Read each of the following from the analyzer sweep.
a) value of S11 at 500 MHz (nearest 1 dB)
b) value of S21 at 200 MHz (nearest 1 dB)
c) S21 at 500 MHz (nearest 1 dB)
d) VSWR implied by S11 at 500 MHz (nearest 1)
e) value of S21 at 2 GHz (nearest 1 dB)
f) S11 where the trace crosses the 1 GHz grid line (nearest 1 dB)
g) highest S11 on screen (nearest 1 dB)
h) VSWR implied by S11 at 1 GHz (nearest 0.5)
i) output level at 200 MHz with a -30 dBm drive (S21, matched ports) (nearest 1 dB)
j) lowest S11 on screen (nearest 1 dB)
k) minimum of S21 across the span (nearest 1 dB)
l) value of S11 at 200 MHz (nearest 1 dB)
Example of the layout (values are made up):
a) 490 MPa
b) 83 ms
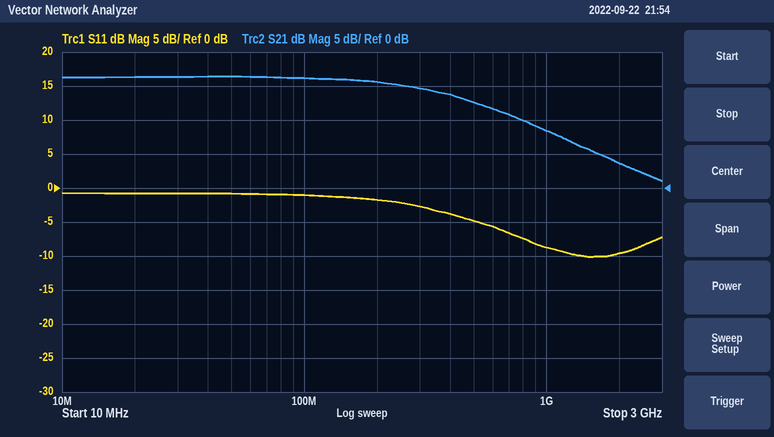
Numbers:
a) -5 dB
b) 16 dB
c) 13 dB
d) 4
e) 4 dB
f) -9 dB
g) -1 dB
h) 2.0
i) -14 dBm
j) -10 dB
k) 1 dB
l) -2 dB
